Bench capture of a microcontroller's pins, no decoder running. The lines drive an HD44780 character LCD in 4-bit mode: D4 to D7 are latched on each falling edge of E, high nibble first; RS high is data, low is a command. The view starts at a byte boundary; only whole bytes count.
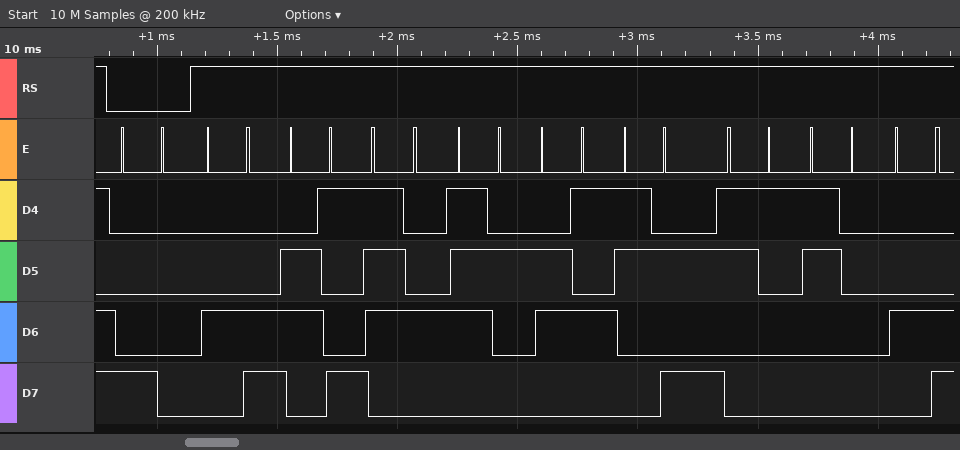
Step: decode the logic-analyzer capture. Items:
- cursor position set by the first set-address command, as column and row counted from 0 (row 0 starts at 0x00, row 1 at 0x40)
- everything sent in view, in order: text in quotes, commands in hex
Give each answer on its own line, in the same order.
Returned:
column 0, row 0
0x80 "Litre:10L"
